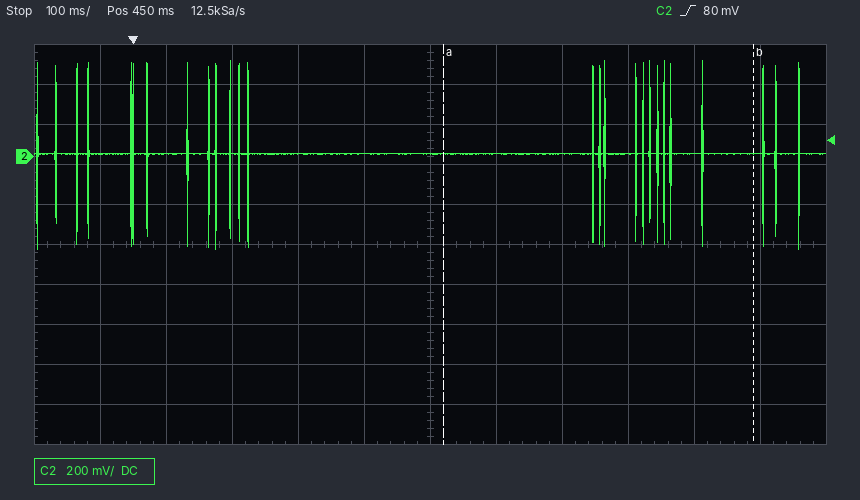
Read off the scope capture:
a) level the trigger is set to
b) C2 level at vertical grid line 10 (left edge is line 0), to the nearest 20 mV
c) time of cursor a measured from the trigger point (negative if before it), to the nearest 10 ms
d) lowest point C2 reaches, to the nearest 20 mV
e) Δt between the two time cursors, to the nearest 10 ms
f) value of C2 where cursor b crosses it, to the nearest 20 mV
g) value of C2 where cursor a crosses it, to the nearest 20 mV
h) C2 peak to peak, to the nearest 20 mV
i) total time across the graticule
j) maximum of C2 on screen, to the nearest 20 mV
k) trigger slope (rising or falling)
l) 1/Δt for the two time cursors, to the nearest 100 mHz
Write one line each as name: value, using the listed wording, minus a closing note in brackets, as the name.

level the trigger is set to: 80 mV
C2 level at vertical grid line 10 (left edge is line 0), to the nearest 20 mV: 20 mV
time of cursor a measured from the trigger point (negative if before it), to the nearest 10 ms: +470 ms
lowest point C2 reaches, to the nearest 20 mV: -460 mV
Δt between the two time cursors, to the nearest 10 ms: 470 ms
value of C2 where cursor b crosses it, to the nearest 20 mV: 20 mV
value of C2 where cursor a crosses it, to the nearest 20 mV: 20 mV
C2 peak to peak, to the nearest 20 mV: 940 mV
total time across the graticule: 1.2 s
maximum of C2 on screen, to the nearest 20 mV: 480 mV
trigger slope: rising
1/Δt for the two time cursors, to the nearest 100 mHz: 2.1 Hz
